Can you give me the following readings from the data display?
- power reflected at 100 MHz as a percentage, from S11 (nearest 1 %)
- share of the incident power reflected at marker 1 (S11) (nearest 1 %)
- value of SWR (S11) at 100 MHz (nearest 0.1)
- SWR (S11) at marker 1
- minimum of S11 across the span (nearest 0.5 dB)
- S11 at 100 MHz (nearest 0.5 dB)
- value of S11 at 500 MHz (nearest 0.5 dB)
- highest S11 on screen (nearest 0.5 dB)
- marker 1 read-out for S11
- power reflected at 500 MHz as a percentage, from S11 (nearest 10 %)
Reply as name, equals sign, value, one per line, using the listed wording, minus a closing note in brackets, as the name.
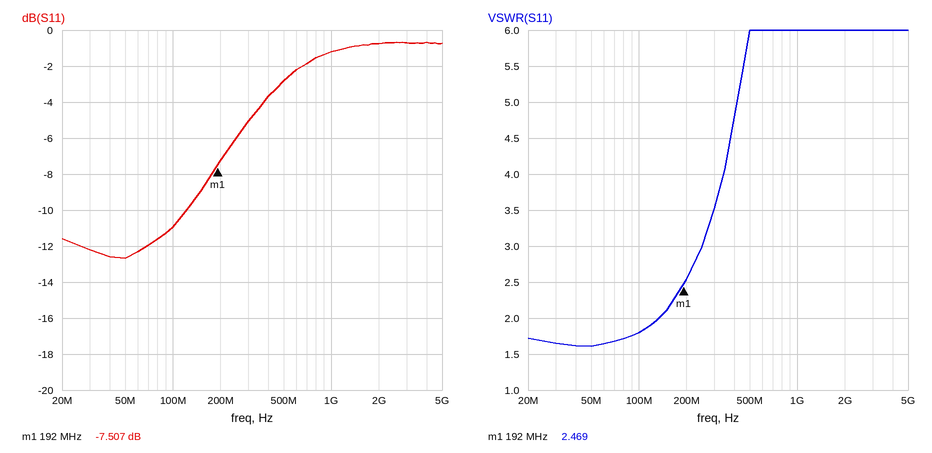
power reflected at 100 MHz as a percentage, from S11 = 8 %
share of the incident power reflected at marker 1 (S11) = 18 %
value of SWR (S11) at 100 MHz = 1.8
SWR (S11) at marker 1 = 2.469
minimum of S11 across the span = -12.5 dB
S11 at 100 MHz = -11.0 dB
value of S11 at 500 MHz = -3.0 dB
highest S11 on screen = -0.5 dB
marker 1 read-out for S11 = -7.507 dB
power reflected at 500 MHz as a percentage, from S11 = 50 %
